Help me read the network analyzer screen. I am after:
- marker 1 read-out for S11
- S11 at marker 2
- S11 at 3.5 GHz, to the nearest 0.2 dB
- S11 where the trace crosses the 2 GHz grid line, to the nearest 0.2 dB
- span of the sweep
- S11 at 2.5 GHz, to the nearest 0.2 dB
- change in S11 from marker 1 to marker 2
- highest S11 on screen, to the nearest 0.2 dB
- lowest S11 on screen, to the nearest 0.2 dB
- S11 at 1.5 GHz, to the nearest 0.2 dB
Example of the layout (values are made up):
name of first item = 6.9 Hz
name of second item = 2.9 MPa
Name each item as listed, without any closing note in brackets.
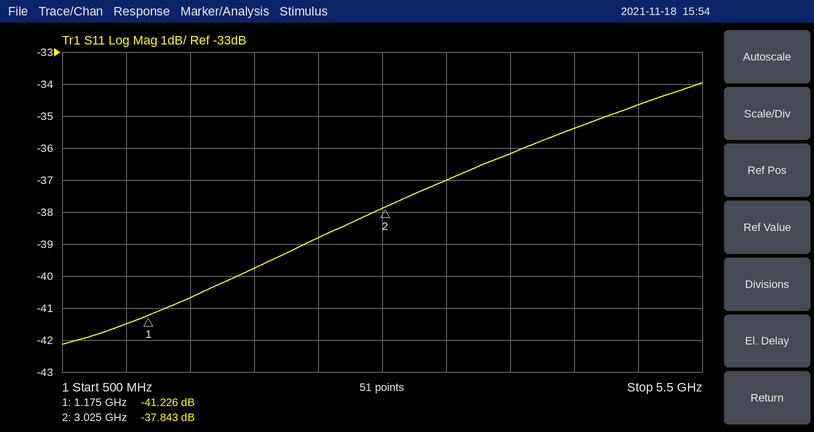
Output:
marker 1 read-out for S11 = -41.226 dB
S11 at marker 2 = -37.843 dB
S11 at 3.5 GHz, to the nearest 0.2 dB = -37.0 dB
S11 where the trace crosses the 2 GHz grid line, to the nearest 0.2 dB = -39.8 dB
span of the sweep = 5 GHz
S11 at 2.5 GHz, to the nearest 0.2 dB = -38.8 dB
change in S11 from marker 1 to marker 2 = 3.383 dB
highest S11 on screen, to the nearest 0.2 dB = -34.0 dB
lowest S11 on screen, to the nearest 0.2 dB = -42.2 dB
S11 at 1.5 GHz, to the nearest 0.2 dB = -40.6 dB
